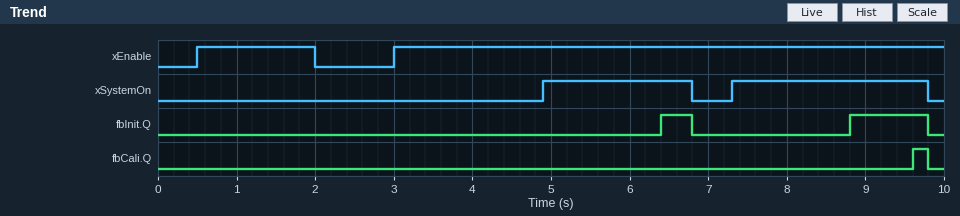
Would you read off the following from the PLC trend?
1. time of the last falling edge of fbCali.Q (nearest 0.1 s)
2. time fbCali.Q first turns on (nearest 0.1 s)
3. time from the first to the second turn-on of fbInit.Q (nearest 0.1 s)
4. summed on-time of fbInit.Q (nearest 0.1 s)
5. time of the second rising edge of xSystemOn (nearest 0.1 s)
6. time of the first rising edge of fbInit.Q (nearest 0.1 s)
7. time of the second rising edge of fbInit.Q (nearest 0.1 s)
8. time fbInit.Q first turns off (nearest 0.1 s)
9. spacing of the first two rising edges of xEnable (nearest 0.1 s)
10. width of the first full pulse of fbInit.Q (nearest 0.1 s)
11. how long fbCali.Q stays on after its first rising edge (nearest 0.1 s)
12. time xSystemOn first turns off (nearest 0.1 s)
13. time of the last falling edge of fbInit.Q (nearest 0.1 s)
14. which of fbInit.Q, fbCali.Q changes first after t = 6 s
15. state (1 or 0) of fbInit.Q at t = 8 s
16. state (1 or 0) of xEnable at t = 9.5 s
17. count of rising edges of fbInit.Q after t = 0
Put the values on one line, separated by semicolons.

9.8 s; 9.6 s; 2.4 s; 1.4 s; 7.3 s; 6.4 s; 8.8 s; 6.8 s; 2.5 s; 0.4 s; 0.2 s; 6.8 s; 9.8 s; fbInit.Q; 0; 1; 2
